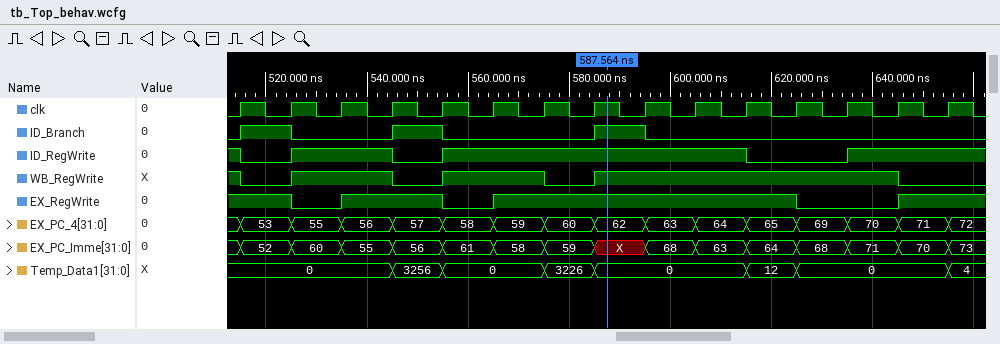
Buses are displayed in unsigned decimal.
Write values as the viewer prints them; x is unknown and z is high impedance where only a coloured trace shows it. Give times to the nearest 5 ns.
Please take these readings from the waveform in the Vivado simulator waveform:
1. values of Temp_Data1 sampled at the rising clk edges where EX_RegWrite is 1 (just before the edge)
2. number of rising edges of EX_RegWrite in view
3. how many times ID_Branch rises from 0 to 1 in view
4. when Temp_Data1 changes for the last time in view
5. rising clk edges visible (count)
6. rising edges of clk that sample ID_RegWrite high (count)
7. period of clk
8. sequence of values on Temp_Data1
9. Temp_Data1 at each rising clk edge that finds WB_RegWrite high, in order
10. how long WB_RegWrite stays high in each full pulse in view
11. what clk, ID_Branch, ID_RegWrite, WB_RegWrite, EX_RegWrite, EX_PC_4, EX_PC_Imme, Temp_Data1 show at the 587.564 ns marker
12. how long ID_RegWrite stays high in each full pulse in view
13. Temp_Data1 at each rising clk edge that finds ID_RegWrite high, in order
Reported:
0, 0, 0, 3256, 0, 3226, 0, 0, 0, 12, 0
3
3
655 ns
15
11
10 ns
0, 3256, 0, 3226, 0, 12, 0, 4
0, 0, 0, 0, 0, 0, 0, 0, 12, 0, 0
20 ns, 20 ns, 60 ns
clk=1, ID_Branch=1, ID_RegWrite=1, WB_RegWrite=1, EX_RegWrite=1, EX_PC_4=62, EX_PC_Imme=X, Temp_Data1=0
20 ns, 60 ns
0, 0, 0, 0, 0, 3226, 0, 0, 0, 0, 0
